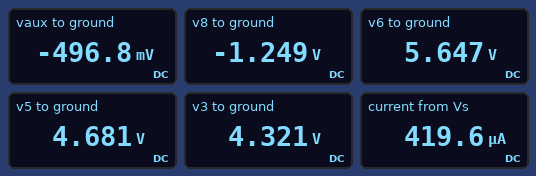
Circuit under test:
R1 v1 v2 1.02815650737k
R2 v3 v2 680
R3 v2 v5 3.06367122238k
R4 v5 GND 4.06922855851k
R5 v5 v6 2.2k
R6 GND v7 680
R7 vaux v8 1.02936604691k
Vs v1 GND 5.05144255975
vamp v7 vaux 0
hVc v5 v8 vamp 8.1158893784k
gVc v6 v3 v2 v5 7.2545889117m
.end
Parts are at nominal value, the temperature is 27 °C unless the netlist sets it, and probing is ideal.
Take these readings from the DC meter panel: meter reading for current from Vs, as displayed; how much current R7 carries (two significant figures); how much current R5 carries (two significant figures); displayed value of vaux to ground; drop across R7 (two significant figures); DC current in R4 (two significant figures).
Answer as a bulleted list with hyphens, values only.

- 419.6 µA
- 730 µA
- 440 µA
- -496.8 mV
- 750 mV
- 1.2 mA
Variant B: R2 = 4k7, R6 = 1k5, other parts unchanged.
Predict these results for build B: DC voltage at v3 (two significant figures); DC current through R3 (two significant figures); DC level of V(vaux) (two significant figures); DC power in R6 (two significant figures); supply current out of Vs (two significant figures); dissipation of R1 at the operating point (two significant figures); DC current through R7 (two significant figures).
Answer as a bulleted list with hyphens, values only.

- 3.2 V
- 15 µA
- -1.3 V
- 1.1 mW
- 320 µA
- 100 µW
- 850 µA
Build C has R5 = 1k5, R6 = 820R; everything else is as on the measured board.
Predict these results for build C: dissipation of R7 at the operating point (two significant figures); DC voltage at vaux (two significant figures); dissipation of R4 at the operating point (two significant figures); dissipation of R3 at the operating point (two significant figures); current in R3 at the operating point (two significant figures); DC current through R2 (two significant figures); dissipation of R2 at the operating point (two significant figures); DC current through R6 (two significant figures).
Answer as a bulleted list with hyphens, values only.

- 580 µW
- -610 mV
- 5.4 mW
- 1.1 µW
- 19 µA
- 420 µA
- 120 µW
- 750 µA
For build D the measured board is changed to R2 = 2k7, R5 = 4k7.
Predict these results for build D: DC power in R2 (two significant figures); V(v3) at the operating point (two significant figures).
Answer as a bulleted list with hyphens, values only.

- 520 µW
- 3.4 V
